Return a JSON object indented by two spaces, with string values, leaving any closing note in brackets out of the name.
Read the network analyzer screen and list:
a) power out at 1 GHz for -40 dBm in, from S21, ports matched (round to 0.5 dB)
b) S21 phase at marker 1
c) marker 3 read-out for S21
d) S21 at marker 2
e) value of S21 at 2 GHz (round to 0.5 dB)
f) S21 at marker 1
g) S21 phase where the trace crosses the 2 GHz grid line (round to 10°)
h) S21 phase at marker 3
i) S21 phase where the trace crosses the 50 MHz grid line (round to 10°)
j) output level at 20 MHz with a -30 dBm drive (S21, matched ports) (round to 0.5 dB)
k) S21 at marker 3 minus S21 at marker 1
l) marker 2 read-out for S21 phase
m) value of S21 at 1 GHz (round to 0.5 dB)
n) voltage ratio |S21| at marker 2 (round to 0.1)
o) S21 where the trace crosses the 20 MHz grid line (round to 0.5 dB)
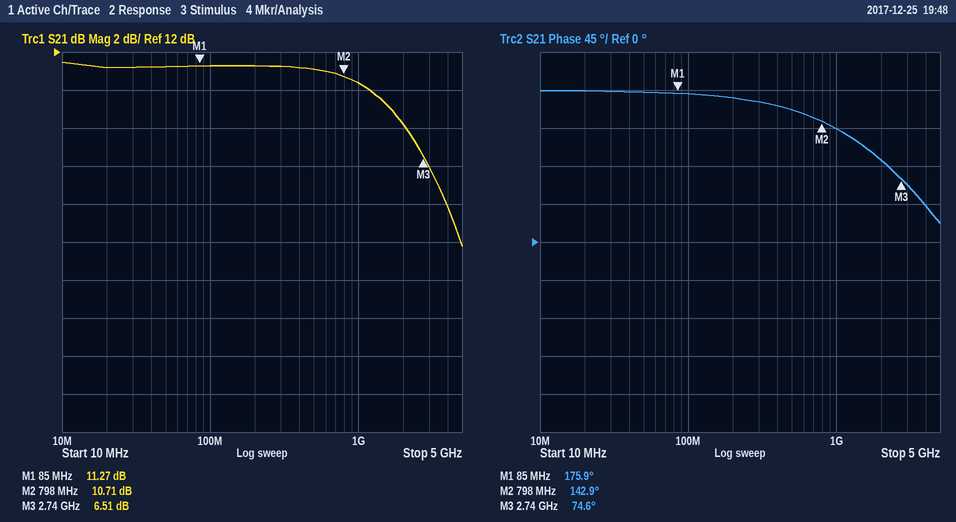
{
  "power out at 1 GHz for -40 dBm in, from S21, ports matched": "-29.5 dBm",
  "S21 phase at marker 1": "175.9°",
  "marker 3 read-out for S21": "6.51 dB",
  "S21 at marker 2": "10.71 dB",
  "value of S21 at 2 GHz": "8.0 dB",
  "S21 at marker 1": "11.27 dB",
  "S21 phase where the trace crosses the 2 GHz grid line": "100°",
  "S21 phase at marker 3": "74.6°",
  "S21 phase where the trace crosses the 50 MHz grid line": "180°",
  "output level at 20 MHz with a -30 dBm drive (S21, matched ports)": "-19.0 dBm",
  "S21 at marker 3 minus S21 at marker 1": "-4.76 dB",
  "marker 2 read-out for S21 phase": "142.9°",
  "value of S21 at 1 GHz": "10.5 dB",
  "voltage ratio |S21| at marker 2": "3.4",
  "S21 where the trace crosses the 20 MHz grid line": "11.0 dB"
}
